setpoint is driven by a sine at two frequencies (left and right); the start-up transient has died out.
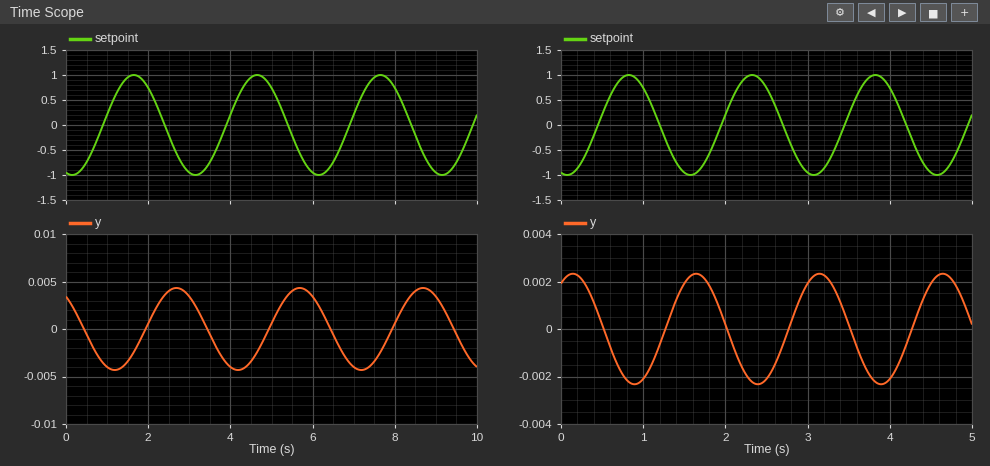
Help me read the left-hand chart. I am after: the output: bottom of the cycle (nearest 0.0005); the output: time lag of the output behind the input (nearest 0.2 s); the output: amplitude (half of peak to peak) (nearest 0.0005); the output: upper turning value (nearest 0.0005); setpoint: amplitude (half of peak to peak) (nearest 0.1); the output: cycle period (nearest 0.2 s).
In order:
-0.0045
1.0 s
0.0045
0.0045
1.0
3.0 s
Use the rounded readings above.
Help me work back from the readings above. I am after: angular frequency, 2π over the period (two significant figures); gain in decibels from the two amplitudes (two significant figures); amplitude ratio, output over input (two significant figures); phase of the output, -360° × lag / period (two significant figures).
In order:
2.1 rad/s
-47 dB
0.0045
-120°
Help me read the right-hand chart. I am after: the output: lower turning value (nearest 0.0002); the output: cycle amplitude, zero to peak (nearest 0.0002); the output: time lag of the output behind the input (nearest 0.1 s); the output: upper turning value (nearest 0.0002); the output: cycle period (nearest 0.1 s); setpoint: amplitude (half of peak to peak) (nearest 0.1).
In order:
-0.0024
0.0024
0.8 s
0.0024
1.5 s
1.0
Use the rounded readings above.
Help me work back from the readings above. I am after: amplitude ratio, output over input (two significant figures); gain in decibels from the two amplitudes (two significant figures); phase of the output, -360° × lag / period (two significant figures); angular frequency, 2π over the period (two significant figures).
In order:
0.0024
-52 dB
-190°
4.2 rad/s
